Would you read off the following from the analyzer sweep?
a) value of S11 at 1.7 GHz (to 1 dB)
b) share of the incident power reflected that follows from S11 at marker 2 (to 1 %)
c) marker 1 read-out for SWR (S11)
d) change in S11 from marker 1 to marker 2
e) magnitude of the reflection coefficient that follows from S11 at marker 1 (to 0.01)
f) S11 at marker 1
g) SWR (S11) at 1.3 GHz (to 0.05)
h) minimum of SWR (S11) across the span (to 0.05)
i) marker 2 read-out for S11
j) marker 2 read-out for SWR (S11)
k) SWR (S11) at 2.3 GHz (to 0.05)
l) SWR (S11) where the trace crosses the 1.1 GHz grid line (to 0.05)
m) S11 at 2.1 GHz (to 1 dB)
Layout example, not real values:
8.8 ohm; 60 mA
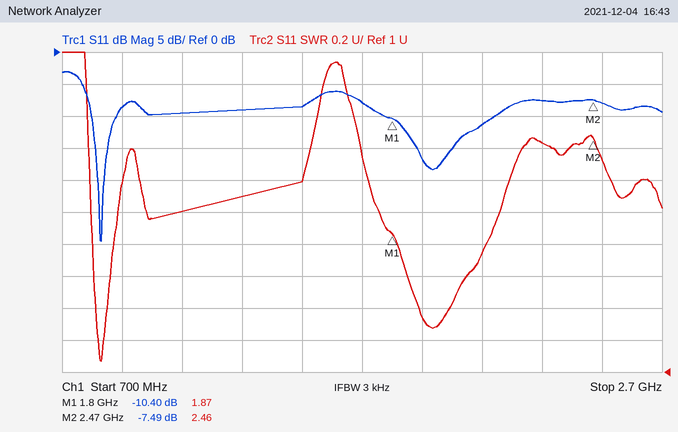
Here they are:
-8 dB; 18 %; 1.87; 2.91 dB; 0.30; -10.40 dB; 2.10; 1.05; -7.49 dB; 2.46; 2.45; 2.00; -11 dB
